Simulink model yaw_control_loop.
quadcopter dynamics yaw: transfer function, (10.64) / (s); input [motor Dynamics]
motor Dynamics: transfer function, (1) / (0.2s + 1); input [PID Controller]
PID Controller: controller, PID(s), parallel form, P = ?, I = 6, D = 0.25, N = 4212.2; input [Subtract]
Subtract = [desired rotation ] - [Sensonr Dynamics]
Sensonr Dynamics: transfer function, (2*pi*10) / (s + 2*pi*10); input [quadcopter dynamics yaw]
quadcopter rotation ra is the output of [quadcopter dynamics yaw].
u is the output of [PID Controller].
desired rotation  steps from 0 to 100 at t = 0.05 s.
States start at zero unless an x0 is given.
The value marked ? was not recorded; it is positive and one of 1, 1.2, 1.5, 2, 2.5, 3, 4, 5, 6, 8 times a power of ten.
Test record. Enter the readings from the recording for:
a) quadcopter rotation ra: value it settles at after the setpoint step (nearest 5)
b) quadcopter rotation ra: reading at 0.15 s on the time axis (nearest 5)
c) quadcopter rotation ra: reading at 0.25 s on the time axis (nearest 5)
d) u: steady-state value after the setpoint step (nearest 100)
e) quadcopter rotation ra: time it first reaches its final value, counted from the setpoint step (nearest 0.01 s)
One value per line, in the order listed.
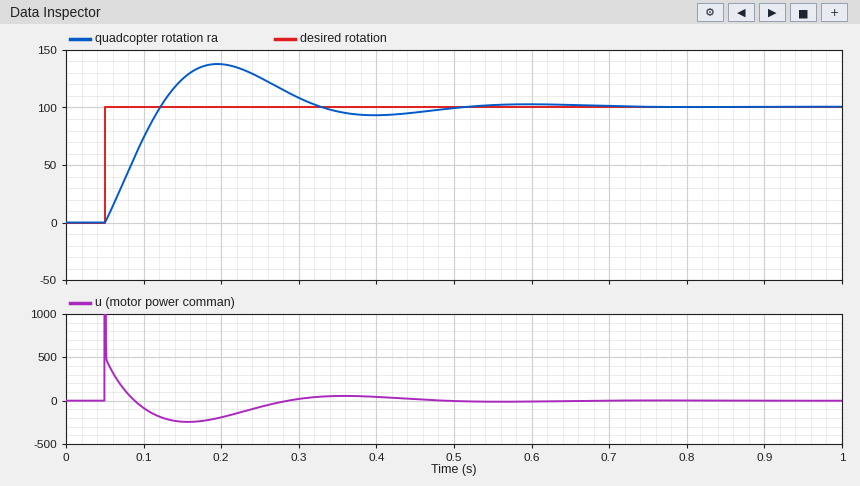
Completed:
100
125
125
0
0.07 s
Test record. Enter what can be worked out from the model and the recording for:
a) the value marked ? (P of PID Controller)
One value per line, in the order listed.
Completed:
5
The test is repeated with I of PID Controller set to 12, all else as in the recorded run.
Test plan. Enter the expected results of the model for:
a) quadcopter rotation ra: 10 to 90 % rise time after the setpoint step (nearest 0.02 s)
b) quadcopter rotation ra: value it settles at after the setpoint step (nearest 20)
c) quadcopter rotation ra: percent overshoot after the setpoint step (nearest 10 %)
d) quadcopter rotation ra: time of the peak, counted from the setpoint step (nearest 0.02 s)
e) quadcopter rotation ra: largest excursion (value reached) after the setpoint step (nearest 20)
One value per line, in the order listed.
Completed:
0.06 s
100
40 %
0.14 s
140
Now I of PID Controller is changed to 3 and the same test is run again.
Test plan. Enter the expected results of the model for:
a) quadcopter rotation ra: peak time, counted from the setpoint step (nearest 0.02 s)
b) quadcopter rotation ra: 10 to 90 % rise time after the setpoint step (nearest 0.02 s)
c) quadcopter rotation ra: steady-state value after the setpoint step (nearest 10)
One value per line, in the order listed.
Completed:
0.14 s
0.06 s
100
